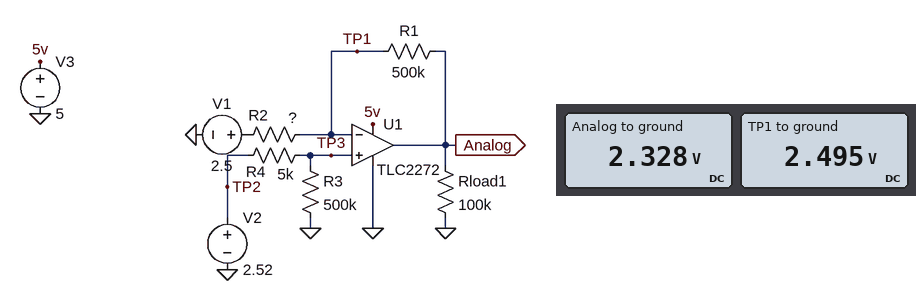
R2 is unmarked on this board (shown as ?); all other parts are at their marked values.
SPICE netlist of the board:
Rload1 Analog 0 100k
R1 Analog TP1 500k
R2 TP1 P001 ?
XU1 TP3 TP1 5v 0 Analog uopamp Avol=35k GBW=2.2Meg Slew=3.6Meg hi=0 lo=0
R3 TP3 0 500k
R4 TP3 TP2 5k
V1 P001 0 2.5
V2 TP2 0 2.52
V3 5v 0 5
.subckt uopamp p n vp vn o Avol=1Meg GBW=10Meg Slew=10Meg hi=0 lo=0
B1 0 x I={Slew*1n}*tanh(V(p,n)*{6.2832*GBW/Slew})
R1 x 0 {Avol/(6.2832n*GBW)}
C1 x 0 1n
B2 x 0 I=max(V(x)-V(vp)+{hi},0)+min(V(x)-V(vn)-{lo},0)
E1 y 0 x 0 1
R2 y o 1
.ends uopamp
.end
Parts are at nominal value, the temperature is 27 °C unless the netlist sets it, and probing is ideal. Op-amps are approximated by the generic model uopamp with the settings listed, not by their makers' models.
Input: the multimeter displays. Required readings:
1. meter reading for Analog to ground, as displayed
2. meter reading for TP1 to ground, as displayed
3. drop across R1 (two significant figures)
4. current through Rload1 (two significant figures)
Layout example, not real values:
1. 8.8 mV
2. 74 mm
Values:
1. 2.328 V
2. 2.495 V
3. 170 mV
4. 23 µA
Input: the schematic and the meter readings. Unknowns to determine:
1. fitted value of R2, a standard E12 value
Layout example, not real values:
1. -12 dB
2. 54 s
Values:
1. 15 kΩ
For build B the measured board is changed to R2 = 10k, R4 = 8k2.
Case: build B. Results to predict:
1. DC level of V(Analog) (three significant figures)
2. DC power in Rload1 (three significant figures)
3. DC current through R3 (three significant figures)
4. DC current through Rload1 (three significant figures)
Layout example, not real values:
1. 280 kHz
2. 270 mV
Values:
1. 1.44 V
2. 20.9 µW
3. 4.96 µA
4. 14.4 µA
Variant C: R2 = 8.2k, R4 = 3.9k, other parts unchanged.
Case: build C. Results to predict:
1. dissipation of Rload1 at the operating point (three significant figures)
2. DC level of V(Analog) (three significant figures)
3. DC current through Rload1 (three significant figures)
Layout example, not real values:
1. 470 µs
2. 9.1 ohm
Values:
1. 63.8 µW
2. 2.53 V
3. 25.3 µA
